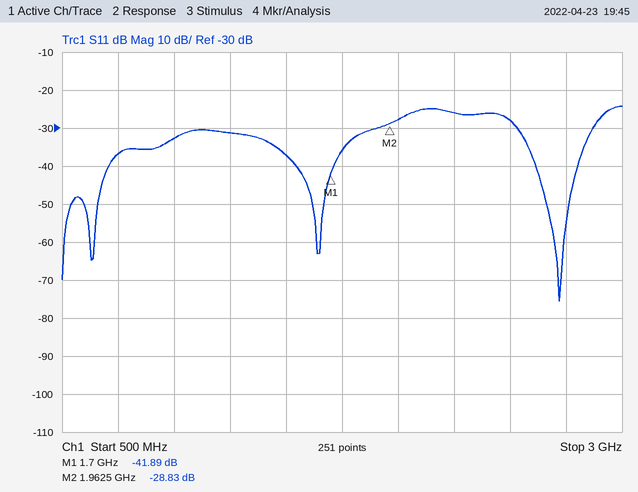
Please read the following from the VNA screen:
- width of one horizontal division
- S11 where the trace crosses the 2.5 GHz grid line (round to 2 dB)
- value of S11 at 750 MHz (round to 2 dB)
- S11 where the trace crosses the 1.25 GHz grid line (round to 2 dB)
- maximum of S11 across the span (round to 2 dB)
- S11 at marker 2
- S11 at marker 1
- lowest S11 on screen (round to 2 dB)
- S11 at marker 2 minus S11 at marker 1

250 MHz
-28 dB
-36 dB
-32 dB
-24 dB
-28.83 dB
-41.89 dB
-76 dB
13.06 dB
